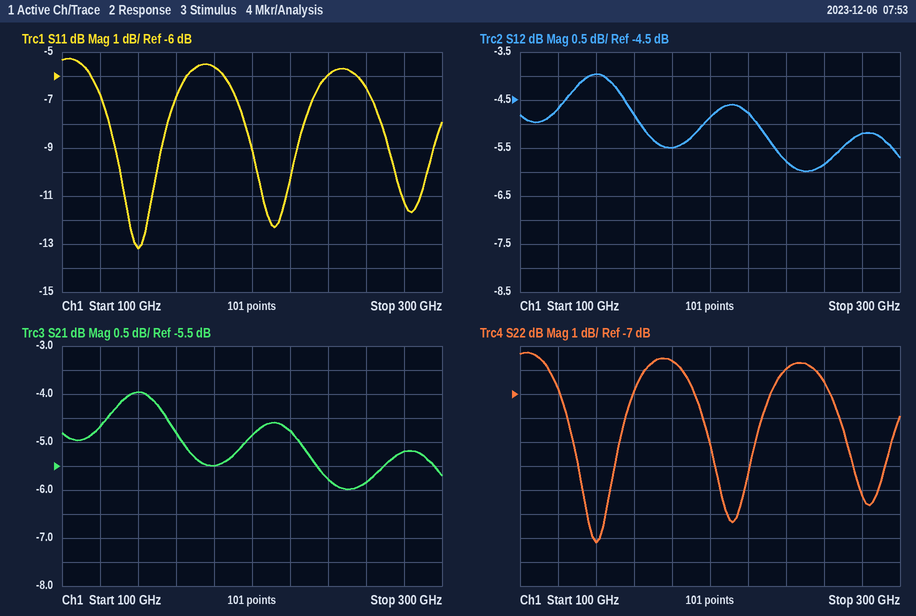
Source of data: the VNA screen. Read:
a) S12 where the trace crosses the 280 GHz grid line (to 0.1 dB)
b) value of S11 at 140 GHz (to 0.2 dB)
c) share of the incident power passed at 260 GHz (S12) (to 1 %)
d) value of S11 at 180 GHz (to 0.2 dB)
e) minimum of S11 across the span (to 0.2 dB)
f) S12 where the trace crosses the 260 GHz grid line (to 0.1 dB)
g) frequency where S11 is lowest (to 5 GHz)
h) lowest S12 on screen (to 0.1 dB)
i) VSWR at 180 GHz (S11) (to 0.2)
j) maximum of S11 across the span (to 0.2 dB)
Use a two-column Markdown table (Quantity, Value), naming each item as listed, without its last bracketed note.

| Quantity | Value |
|---|---|
| S12 where the trace crosses the 280 GHz grid line | -5.2 dB |
| value of S11 at 140 GHz | -13.2 dB |
| share of the incident power passed at 260 GHz (S12) | 26 % |
| value of S11 at 180 GHz | -5.6 dB |
| minimum of S11 across the span | -13.2 dB |
| S12 where the trace crosses the 260 GHz grid line | -5.8 dB |
| frequency where S11 is lowest | 140 GHz |
| lowest S12 on screen | -6.0 dB |
| VSWR at 180 GHz (S11) | 3.2 |
| maximum of S11 across the span | -5.2 dB |
